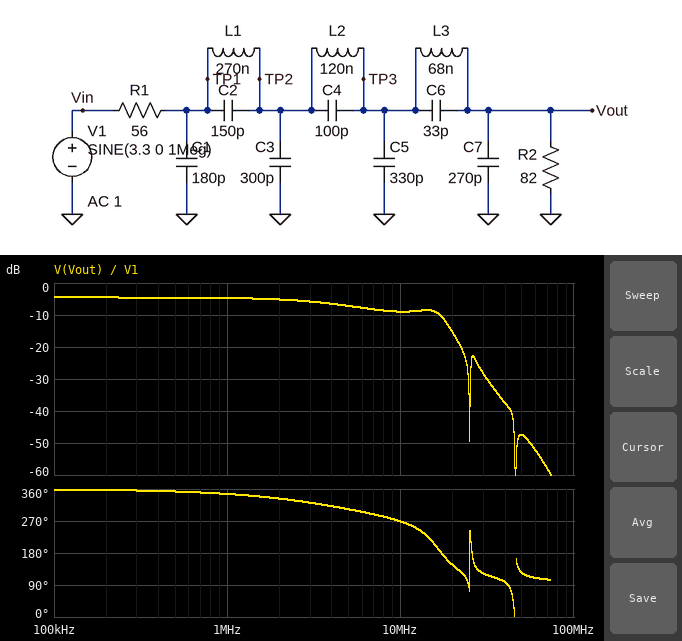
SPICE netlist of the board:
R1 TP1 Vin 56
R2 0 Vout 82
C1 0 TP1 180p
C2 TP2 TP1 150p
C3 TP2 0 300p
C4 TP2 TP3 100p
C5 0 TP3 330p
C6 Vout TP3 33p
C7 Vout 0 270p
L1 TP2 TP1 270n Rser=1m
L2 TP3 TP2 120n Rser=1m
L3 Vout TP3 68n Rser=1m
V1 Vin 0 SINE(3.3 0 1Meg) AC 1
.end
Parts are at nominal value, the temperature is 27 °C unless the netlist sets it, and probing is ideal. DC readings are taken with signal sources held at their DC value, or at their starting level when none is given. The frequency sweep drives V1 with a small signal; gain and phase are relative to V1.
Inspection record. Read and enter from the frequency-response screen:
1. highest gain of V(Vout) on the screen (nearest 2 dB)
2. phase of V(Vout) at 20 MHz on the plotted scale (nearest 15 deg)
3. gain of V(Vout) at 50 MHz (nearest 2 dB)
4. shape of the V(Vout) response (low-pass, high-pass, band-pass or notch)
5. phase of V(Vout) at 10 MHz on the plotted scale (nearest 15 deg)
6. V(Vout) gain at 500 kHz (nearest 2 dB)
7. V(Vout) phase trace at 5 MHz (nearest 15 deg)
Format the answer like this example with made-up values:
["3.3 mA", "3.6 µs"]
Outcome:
["-4 dB", "150 deg", "-48 dB", "low-pass", "270 deg", "-4 dB", "300 deg"]
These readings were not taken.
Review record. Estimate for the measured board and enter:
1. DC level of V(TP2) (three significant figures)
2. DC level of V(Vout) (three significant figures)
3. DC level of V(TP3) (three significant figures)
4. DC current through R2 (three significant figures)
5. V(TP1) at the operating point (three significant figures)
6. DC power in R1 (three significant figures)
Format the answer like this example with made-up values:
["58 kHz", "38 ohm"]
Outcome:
["1.96 V", "1.96 V", "1.96 V", "23.9 mA", "1.96 V", "32.0 mW"]
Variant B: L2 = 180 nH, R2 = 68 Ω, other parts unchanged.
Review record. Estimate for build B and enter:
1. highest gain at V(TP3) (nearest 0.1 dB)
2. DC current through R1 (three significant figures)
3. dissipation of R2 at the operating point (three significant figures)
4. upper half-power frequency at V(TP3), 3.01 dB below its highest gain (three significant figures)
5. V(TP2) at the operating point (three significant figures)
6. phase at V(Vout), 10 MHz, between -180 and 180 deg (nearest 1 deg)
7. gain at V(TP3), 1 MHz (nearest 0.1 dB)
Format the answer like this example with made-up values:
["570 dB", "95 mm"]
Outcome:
["-5.2 dB", "26.6 mA", "48.2 mW", "6.29 MHz", "1.81 V", "-94 deg", "-5.4 dB"]
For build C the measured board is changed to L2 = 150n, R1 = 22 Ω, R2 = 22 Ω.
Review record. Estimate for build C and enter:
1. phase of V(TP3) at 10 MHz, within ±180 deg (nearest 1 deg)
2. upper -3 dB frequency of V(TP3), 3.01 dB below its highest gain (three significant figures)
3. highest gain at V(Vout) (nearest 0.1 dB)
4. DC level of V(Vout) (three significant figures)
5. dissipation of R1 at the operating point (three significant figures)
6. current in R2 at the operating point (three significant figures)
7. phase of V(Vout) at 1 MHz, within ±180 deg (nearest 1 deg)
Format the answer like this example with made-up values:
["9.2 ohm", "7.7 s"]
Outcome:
["-79 deg", "13.5 MHz", "-6.0 dB", "1.65 V", "124 mW", "75.0 mA", "-8 deg"]
